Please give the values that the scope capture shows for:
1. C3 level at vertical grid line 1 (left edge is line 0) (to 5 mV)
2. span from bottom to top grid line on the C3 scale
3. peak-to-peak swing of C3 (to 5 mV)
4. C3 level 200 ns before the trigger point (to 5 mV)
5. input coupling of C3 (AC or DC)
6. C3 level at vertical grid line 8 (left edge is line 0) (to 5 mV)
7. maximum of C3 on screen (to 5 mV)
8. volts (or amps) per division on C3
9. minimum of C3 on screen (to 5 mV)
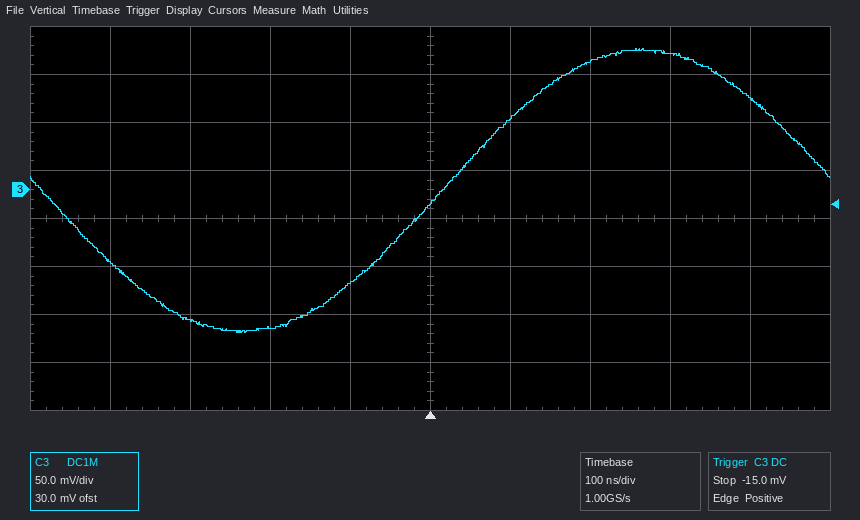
-75 mV
400 mV
295 mV
-145 mV
DC
140 mV
145 mV
50 mV
-150 mV
